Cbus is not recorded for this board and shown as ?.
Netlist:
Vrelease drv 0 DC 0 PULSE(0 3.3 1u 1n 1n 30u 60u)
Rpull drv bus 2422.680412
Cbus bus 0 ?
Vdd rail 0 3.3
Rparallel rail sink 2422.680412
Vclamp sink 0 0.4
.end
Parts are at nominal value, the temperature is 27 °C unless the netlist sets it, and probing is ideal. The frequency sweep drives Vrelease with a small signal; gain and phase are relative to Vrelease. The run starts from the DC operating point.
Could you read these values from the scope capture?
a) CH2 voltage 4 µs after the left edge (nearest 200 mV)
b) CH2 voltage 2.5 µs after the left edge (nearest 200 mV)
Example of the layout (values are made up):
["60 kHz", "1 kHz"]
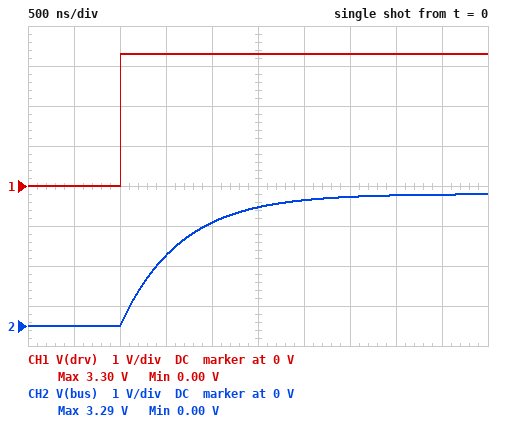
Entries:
["3.2 V", "3.0 V"]
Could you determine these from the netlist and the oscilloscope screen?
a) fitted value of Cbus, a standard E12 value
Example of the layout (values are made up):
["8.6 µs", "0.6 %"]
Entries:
["270 pF"]
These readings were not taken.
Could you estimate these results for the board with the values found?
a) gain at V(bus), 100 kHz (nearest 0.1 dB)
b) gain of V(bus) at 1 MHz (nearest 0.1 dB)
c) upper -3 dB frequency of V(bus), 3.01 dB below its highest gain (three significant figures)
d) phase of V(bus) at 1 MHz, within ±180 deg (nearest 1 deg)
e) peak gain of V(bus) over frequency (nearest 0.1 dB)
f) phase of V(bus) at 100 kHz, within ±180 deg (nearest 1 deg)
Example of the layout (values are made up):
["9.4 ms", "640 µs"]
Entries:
["-0.7 dB", "-12.5 dB", "243 kHz", "-76 deg", "0 dB", "-22 deg"]
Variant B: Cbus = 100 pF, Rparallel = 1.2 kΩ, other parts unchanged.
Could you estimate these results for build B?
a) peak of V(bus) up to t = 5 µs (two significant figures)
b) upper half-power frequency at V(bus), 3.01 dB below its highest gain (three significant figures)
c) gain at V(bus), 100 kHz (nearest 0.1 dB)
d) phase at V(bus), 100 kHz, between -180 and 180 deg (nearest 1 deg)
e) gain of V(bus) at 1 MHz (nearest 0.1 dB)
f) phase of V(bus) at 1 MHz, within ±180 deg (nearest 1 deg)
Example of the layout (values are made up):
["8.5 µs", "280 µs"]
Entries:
["3.3 V", "657 kHz", "-0.1 dB", "-9 deg", "-5.2 dB", "-57 deg"]
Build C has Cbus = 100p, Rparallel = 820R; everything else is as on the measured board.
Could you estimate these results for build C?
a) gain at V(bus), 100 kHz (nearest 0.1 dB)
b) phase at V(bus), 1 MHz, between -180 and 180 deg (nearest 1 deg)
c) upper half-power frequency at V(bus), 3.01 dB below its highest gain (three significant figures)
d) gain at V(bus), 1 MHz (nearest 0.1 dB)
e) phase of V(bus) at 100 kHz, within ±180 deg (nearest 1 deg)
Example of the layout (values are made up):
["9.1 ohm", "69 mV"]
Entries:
["-0.1 dB", "-57 deg", "657 kHz", "-5.2 dB", "-9 deg"]
